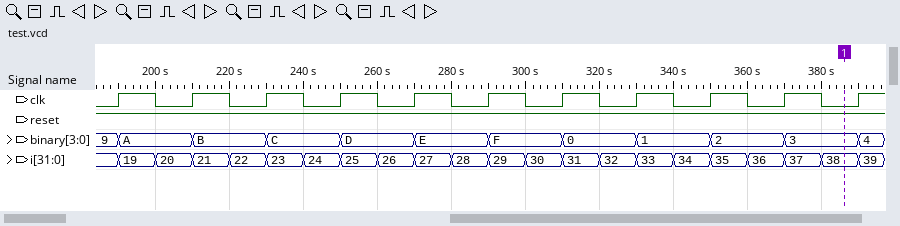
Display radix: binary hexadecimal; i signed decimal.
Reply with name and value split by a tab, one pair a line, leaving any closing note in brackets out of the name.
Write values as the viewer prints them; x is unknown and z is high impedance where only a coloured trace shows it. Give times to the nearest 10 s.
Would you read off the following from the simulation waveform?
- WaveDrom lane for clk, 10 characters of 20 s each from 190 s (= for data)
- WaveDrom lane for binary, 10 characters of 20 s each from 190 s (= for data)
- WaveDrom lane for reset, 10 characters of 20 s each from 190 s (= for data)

WaveDrom lane for clk, 10 characters of 20 s each from 190 s	{name: 'clk', wave: 'p.........'}
WaveDrom lane for binary, 10 characters of 20 s each from 190 s	{name: 'binary', wave: '==========', data: 'A B C D E F 0 1 2 3'}
WaveDrom lane for reset, 10 characters of 20 s each from 190 s	{name: 'reset', wave: '1.........'}
